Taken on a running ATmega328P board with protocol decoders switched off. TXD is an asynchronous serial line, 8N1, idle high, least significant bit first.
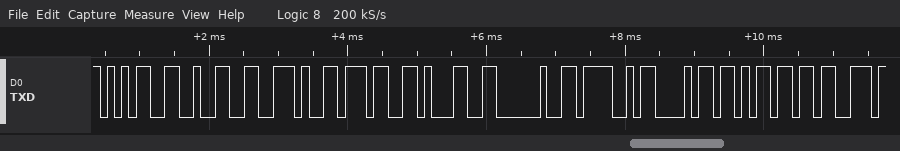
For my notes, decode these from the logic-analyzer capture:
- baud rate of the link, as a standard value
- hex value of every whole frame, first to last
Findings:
9600 baud
0x35 0x32 0x2E 0x37 0x31 0x20 0x4F 0x68 0x6D 0x73
